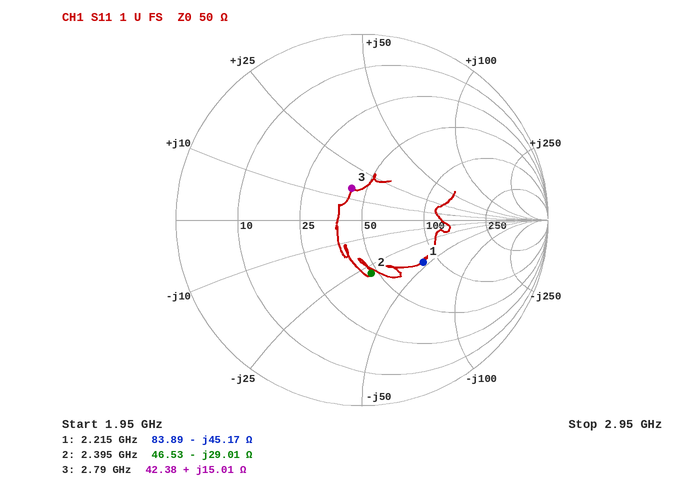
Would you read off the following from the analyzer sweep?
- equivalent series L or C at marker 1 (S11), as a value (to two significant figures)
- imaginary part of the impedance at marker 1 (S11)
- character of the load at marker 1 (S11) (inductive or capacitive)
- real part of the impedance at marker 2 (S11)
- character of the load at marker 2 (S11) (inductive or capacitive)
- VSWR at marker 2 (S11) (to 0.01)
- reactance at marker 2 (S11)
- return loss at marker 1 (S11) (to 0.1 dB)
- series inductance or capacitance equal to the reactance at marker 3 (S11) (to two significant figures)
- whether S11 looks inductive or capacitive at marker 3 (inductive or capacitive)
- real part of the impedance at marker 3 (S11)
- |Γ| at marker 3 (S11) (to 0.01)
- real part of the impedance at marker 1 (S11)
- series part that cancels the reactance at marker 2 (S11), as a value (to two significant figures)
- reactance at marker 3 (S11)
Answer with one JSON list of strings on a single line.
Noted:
["1.6 pF", "-45.17 Ω", "capacitive", "46.53 Ω", "capacitive", "1.82", "-29.01 Ω", "8.0 dB", "860 pH", "inductive", "42.38 Ω", "0.18", "83.89 Ω", "1.9 nH", "+15.01 Ω"]
